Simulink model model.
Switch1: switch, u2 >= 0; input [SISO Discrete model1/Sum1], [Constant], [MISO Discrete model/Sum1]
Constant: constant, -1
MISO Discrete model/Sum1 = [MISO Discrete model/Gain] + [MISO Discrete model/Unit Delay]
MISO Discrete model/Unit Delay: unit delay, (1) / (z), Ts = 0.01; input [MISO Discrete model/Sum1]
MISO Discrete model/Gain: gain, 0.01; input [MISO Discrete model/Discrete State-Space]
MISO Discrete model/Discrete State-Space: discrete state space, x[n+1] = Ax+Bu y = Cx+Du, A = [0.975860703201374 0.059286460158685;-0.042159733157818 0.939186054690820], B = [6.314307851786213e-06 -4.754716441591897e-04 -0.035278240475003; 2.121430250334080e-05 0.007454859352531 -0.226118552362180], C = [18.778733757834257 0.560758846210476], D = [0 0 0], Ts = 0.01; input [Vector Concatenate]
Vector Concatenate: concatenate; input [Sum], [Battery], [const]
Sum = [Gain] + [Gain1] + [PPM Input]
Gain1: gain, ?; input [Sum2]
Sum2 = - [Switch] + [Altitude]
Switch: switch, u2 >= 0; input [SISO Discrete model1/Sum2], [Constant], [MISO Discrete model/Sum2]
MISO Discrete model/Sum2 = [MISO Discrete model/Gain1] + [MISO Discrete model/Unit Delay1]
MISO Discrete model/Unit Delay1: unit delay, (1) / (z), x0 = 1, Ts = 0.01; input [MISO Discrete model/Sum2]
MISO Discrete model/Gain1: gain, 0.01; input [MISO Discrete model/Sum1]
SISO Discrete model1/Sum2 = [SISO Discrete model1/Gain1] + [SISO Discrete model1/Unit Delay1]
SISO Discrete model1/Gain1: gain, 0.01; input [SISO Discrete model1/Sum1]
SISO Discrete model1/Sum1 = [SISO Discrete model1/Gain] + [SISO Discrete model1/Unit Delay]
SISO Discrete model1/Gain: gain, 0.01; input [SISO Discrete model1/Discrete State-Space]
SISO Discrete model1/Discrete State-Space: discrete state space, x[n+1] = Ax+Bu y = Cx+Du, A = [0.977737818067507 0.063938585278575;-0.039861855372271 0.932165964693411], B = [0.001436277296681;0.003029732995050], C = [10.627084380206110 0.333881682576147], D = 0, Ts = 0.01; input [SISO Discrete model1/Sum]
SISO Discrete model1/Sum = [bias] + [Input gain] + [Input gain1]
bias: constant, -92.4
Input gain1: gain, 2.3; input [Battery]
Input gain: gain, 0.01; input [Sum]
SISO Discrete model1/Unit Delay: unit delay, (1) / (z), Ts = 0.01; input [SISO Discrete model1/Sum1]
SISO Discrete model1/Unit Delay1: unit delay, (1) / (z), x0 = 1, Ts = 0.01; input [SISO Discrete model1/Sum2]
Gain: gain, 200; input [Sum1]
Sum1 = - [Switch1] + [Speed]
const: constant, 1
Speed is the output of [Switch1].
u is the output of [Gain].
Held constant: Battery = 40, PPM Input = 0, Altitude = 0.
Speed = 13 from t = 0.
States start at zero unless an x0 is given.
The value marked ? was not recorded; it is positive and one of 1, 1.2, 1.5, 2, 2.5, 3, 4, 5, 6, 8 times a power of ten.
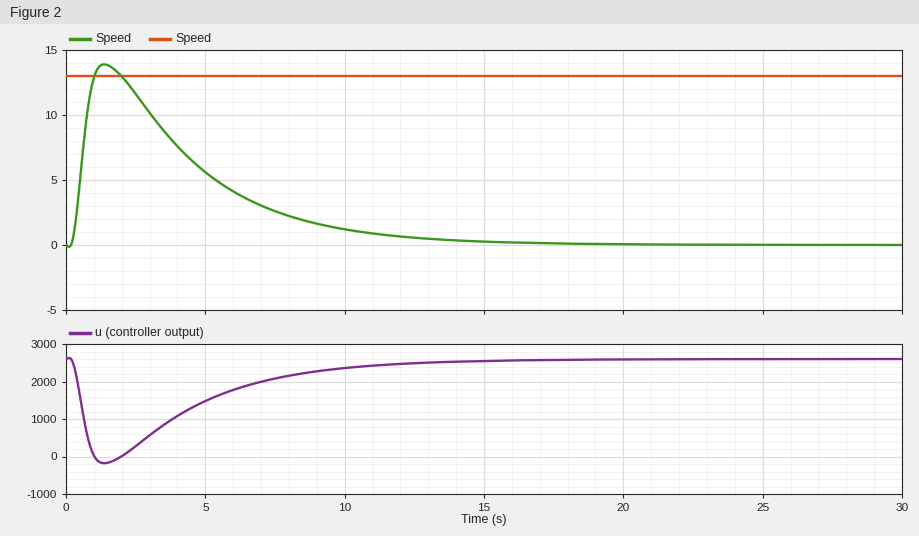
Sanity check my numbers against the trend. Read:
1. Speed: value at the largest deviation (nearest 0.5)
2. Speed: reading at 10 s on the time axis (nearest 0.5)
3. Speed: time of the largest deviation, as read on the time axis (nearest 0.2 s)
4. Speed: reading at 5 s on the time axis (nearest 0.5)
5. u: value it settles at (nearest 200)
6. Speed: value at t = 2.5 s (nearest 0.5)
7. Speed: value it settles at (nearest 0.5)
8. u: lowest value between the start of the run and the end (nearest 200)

14.0
1.0
1.4 s
5.5
2600
11.5
0.0
-200
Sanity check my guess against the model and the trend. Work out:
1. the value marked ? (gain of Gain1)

50
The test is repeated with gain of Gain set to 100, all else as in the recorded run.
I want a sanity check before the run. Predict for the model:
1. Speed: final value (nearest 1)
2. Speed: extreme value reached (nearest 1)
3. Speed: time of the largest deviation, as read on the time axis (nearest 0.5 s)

0
13
2.0 s
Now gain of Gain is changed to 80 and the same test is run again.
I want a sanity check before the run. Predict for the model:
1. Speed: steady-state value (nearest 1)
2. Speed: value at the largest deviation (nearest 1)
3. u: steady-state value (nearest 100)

0
12
1000
